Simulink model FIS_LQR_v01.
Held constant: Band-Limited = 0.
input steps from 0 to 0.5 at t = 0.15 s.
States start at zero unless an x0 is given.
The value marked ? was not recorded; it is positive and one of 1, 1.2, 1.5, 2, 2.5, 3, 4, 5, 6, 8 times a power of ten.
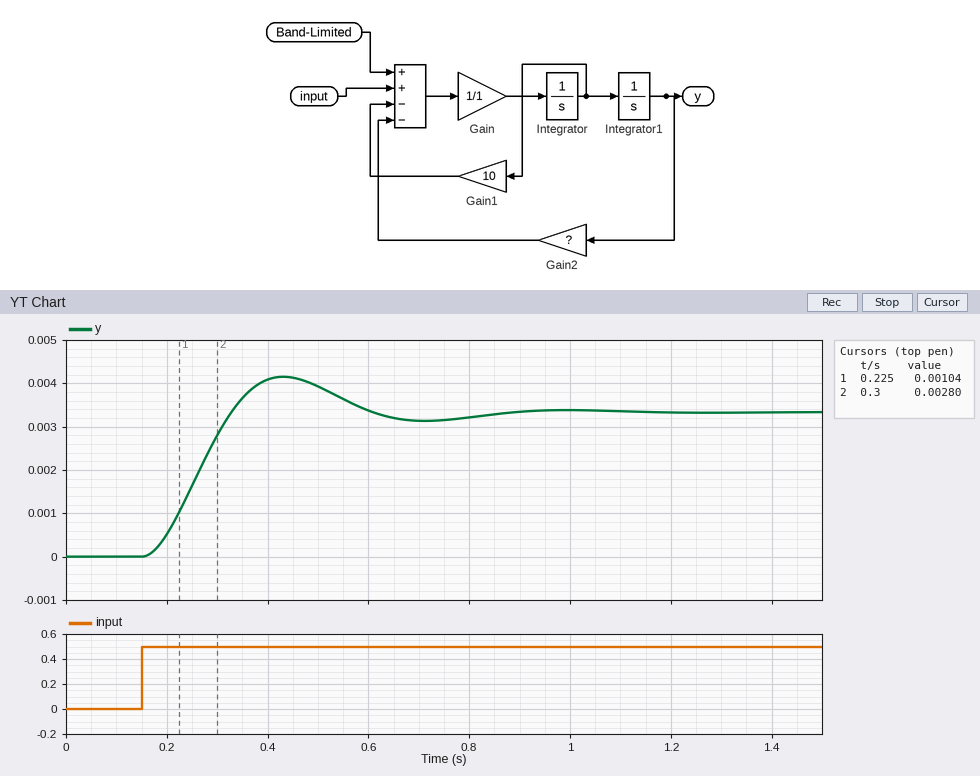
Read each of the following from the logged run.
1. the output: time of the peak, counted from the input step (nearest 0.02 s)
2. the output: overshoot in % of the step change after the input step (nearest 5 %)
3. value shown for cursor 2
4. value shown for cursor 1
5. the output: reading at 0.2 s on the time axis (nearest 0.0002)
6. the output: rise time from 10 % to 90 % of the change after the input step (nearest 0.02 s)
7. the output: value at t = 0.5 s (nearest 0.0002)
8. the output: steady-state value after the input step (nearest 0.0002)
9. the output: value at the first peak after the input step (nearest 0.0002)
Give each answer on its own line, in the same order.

0.28 s
25 %
0.00280
0.00104
0.0006
0.12 s
0.0040
0.0034
0.0042
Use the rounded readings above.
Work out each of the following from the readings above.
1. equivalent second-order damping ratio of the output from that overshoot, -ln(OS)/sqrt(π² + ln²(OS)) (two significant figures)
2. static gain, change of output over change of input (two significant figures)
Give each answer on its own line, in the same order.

0.40
0.0068
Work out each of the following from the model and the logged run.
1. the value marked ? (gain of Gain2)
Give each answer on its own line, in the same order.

150
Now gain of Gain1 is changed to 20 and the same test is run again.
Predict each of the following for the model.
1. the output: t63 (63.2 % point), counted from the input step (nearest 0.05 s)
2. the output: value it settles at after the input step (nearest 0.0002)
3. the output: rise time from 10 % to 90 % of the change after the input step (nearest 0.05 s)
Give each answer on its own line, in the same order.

0.15 s
0.0034
0.20 s
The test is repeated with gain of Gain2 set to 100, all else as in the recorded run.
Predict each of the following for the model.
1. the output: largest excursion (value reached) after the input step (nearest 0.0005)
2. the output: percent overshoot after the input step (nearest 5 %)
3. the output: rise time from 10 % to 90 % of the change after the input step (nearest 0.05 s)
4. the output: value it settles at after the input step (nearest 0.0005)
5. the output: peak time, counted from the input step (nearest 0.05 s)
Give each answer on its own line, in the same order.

0.0060
15 %
0.15 s
0.0050
0.35 s
